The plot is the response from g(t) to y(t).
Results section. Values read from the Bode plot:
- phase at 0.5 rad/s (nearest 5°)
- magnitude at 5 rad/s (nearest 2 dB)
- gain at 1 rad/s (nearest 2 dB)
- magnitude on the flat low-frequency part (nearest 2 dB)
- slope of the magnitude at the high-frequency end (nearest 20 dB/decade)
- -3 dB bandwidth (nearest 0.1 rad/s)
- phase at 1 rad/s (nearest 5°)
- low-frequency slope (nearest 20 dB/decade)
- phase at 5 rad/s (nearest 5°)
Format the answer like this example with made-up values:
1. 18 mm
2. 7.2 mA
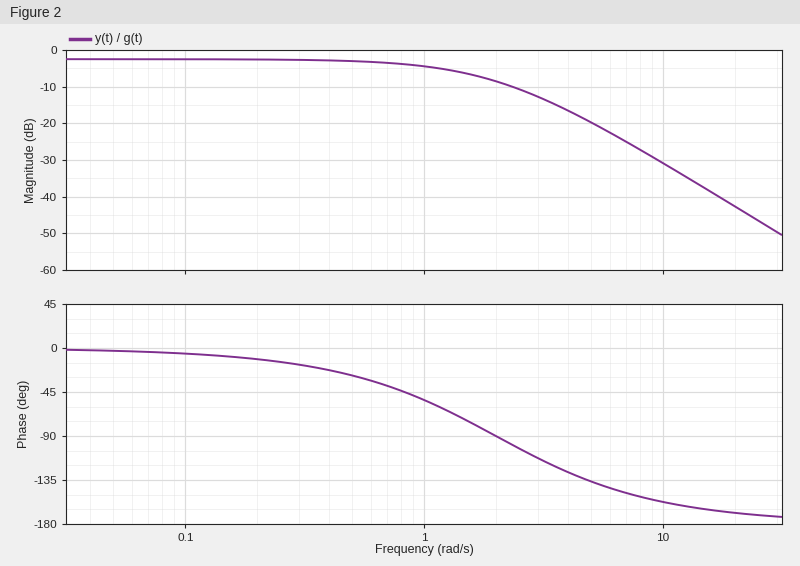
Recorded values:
1. -30°
2. -20 dB
3. -4 dB
4. -2 dB
5. -40 dB/decade
6. 1.3 rad/s
7. -55°
8. 0 dB/decade
9. -135°
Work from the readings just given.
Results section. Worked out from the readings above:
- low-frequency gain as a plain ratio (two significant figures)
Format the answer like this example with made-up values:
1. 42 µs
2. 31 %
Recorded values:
1. 0.79
